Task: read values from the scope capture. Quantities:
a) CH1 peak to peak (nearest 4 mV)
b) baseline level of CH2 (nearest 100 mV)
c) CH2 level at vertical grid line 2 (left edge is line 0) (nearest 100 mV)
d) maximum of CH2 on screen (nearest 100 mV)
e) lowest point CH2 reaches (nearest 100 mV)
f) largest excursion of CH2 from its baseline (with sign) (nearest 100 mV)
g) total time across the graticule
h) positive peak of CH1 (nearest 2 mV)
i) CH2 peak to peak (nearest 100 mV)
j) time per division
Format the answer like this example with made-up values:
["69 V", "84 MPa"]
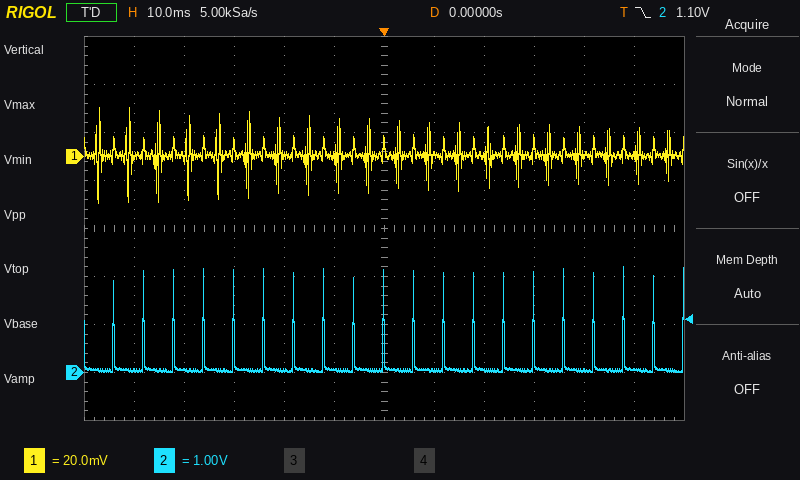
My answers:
["40 mV", "100 mV", "100 mV", "2.2 V", "0.0 V", "+2.1 V", "120 ms", "20 mV", "2.2 V", "10 ms"]
